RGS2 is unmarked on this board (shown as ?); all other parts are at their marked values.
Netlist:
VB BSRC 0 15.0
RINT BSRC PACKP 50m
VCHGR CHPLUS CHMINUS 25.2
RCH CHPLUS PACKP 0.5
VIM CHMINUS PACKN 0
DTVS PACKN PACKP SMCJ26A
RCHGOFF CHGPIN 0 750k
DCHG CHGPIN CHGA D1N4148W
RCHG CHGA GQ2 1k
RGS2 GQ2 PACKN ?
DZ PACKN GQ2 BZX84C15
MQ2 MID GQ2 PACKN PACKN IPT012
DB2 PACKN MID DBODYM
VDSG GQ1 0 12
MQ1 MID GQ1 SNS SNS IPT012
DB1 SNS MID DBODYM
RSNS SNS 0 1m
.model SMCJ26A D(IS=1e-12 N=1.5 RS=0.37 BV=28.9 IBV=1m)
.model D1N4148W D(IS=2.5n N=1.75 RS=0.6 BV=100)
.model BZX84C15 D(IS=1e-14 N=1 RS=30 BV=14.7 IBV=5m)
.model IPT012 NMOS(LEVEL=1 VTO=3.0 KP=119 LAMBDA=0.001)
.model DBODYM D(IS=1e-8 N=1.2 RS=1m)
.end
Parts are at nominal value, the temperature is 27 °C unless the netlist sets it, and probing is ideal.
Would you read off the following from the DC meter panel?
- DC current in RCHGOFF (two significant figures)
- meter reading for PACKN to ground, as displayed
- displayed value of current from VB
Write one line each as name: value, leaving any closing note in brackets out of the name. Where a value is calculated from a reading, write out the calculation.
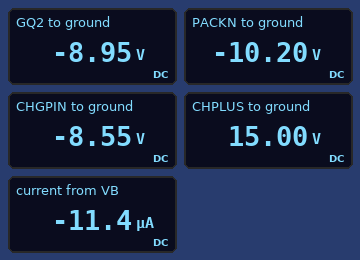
DC current in RCHGOFF: (0 V - (-8.55 V)) / 750 kΩ = 11 µA
meter reading for PACKN to ground, as displayed: -10.20 V
displayed value of current from VB: -11.4 µA
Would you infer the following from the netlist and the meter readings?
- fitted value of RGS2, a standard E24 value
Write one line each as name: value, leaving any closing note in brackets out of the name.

fitted value of RGS2, a standard E24 value: 110 kΩ
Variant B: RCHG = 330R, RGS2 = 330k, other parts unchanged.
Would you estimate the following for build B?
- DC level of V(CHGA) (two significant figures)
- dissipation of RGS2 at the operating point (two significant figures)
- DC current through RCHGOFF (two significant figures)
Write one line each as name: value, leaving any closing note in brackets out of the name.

DC level of V(CHGA): -7.2 V
dissipation of RGS2 at the operating point: 27 µW
DC current through RCHGOFF: 9.1 µA
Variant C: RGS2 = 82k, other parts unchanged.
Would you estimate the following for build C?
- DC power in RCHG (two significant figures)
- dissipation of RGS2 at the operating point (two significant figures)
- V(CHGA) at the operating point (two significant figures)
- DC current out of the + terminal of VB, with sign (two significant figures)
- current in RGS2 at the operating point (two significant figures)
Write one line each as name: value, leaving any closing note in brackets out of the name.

DC power in RCHG: 140 nW
dissipation of RGS2 at the operating point: 11 µW
V(CHGA) at the operating point: -9.2 V
DC current out of the + terminal of VB, with sign: -12 µA
current in RGS2 at the operating point: 12 µA
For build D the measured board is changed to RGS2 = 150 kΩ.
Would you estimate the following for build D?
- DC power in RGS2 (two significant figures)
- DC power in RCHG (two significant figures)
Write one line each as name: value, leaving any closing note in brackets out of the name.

DC power in RGS2: 18 µW
DC power in RCHG: 120 nW
